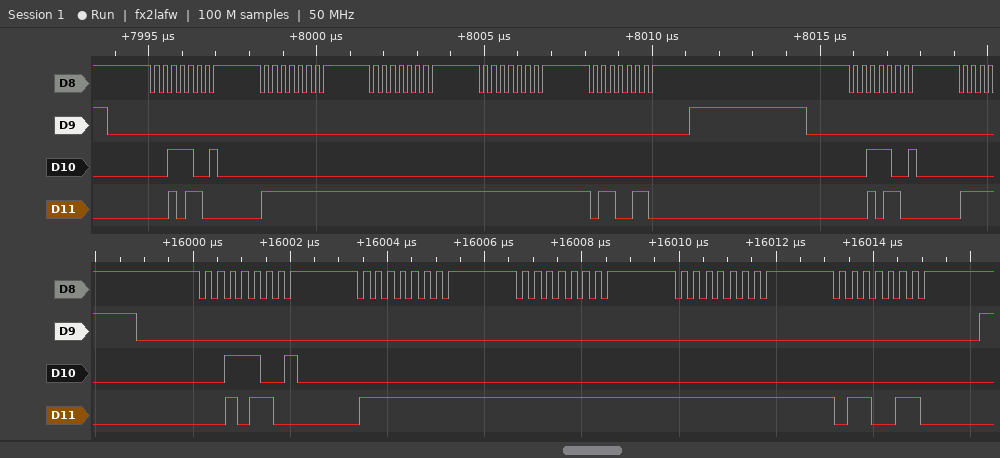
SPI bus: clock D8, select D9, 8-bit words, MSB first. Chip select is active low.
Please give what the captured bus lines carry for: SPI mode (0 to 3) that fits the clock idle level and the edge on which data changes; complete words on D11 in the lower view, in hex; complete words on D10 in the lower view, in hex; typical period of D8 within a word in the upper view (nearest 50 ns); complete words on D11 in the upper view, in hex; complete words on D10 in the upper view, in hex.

3
2C, FF, FF, FF, 66
39, 00, 00, 00, 00
250 ns
2C, FF, FF, FF, 66, 2C
39, 00, 00, 00, 00, 39
